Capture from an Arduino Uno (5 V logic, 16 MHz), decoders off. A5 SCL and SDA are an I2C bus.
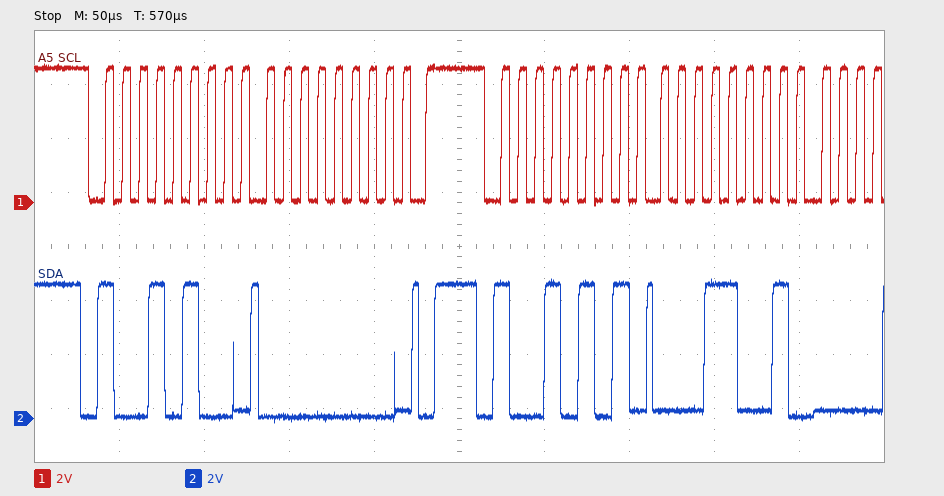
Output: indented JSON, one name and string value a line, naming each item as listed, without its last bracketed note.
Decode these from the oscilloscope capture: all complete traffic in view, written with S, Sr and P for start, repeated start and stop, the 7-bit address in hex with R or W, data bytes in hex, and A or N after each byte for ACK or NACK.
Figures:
{
  "all complete traffic in view, written with S, Sr and P for start, repeated start and stop, the 7-bit address in hex with R or W, data bytes in hex, and A or N after each byte for ACK or NACK": "S 4AW A 00 A P S 4AR A 19 A"
}
